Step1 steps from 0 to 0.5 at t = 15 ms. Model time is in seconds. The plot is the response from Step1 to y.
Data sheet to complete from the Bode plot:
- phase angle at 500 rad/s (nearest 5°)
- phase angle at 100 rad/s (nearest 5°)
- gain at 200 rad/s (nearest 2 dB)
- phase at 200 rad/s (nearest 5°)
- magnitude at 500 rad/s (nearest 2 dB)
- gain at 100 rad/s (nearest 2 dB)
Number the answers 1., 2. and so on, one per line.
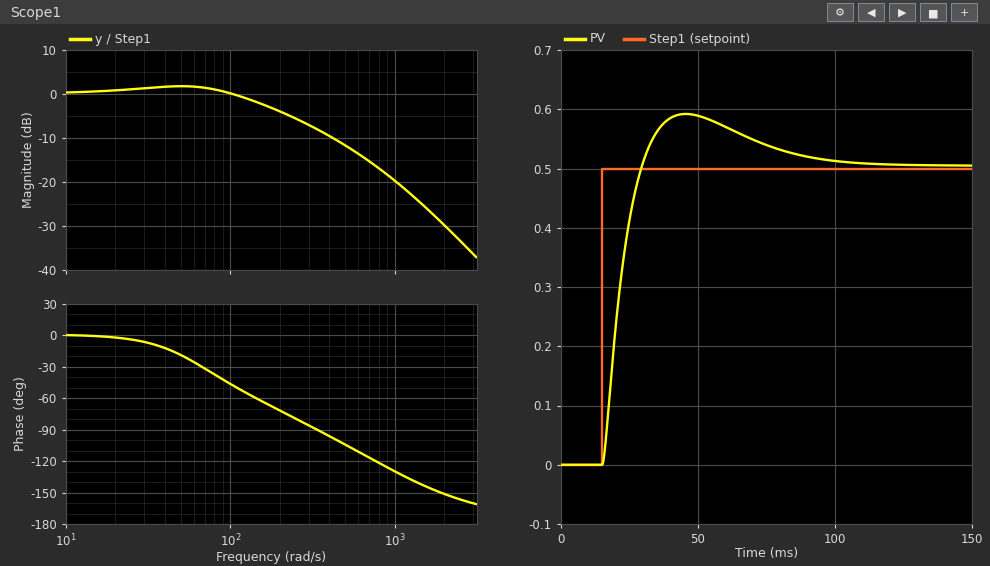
1. -105°
2. -45°
3. -4 dB
4. -70°
5. -12 dB
6. 0 dB
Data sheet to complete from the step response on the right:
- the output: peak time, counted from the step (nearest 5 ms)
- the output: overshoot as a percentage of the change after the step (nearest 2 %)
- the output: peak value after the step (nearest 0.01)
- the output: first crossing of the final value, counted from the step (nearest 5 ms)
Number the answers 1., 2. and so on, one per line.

1. 30 ms
2. 18 %
3. 0.59
4. 15 ms
